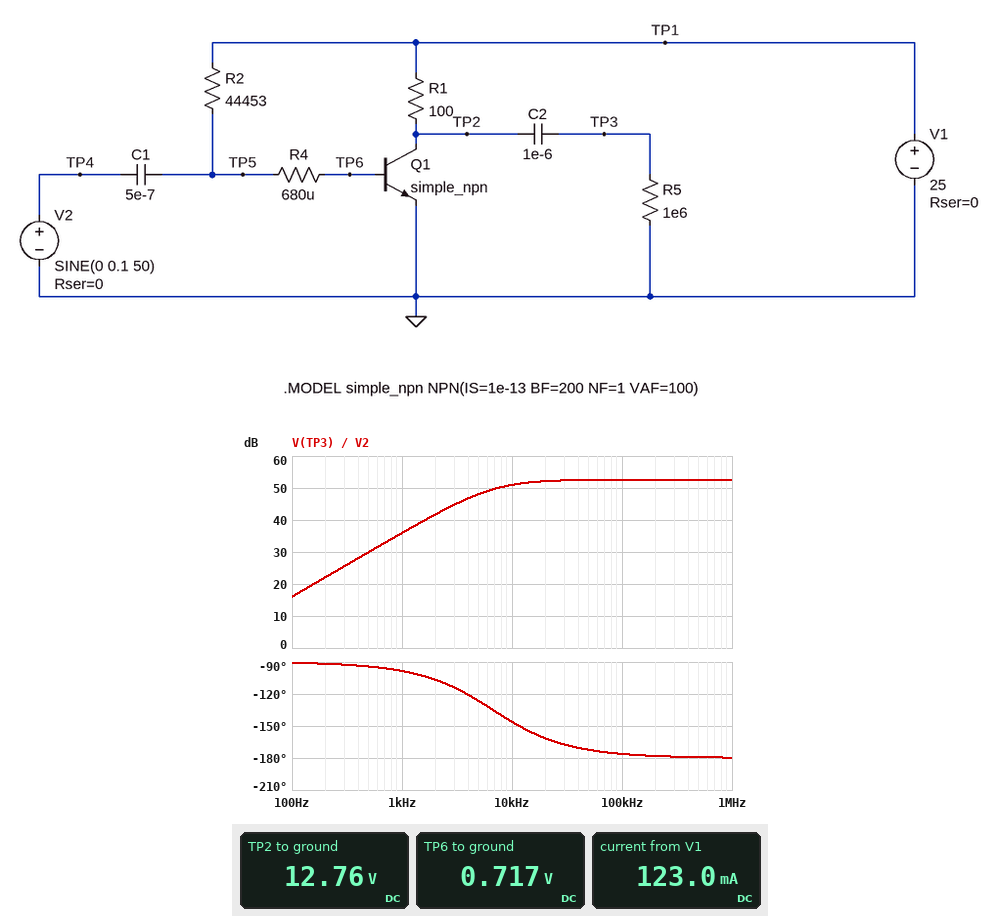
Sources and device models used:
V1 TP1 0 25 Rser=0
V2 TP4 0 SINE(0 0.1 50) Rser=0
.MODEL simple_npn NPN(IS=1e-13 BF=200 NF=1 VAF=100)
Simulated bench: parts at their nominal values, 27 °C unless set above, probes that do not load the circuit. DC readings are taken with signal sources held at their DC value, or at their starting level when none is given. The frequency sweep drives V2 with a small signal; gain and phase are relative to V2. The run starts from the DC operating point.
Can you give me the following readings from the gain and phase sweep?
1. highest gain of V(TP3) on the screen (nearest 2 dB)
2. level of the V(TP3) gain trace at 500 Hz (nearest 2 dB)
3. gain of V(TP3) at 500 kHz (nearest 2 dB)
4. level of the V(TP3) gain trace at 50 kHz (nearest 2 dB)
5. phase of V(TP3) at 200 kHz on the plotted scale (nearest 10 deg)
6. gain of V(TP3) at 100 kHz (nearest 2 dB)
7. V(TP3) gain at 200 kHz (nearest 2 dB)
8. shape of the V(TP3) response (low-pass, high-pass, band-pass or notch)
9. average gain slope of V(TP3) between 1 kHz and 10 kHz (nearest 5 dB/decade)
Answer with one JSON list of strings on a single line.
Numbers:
["52 dB", "30 dB", "52 dB", "52 dB", "-180 deg", "52 dB", "52 dB", "high-pass", "15 dB/decade"]
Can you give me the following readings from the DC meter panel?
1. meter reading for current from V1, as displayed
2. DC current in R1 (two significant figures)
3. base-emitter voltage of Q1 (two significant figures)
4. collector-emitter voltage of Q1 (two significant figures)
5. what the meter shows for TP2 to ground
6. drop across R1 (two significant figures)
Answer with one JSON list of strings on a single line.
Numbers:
["123.0 mA", "120 mA", "720 mV", "13 V", "12.76 V", "12 V"]
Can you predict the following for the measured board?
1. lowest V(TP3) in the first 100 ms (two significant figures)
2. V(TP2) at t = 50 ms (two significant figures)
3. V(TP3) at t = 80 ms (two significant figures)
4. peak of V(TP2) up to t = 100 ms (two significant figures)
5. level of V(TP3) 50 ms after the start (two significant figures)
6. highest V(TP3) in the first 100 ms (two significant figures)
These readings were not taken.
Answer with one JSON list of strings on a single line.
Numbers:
["-320 mV", "13 V", "-320 mV", "13 V", "320 mV", "320 mV"]
